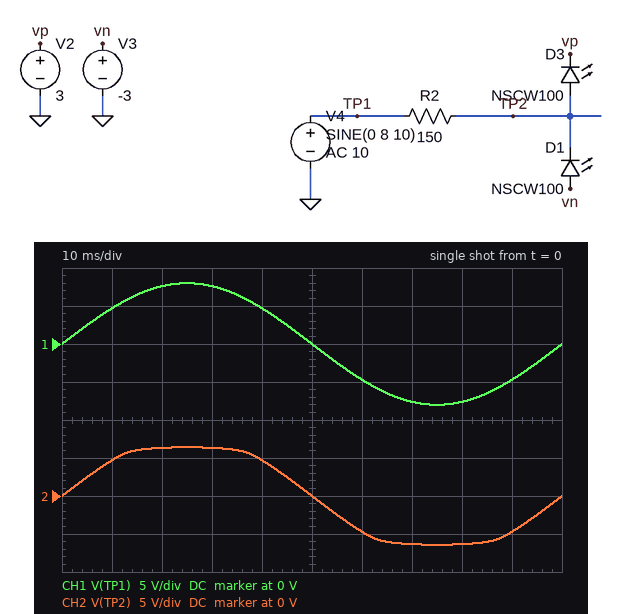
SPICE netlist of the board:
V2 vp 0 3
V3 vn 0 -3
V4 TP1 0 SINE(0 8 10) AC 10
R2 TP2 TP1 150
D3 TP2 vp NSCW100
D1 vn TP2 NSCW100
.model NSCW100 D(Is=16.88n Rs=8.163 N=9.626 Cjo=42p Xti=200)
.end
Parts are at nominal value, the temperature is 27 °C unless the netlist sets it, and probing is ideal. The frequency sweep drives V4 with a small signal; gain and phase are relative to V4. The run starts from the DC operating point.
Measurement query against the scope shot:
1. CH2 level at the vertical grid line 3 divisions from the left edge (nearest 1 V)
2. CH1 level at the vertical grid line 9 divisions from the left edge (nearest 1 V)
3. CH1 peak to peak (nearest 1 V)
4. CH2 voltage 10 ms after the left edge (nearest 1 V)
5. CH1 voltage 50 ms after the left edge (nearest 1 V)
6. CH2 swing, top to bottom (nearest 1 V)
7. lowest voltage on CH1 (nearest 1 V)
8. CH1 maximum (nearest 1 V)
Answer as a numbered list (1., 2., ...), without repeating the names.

1. 6 V
2. -5 V
3. 16 V
4. 5 V
5. 0 V
6. 13 V
7. -8 V
8. 8 V
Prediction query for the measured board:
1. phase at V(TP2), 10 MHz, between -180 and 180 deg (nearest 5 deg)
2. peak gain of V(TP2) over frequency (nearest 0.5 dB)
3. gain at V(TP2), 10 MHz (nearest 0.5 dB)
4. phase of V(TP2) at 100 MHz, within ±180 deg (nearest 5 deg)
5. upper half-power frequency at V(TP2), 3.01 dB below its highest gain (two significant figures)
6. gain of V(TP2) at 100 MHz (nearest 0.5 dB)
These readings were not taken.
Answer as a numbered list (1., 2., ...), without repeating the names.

1. -20 deg
2. 0 dB
3. -0.5 dB
4. -70 deg
5. 25 MHz
6. -12.5 dB
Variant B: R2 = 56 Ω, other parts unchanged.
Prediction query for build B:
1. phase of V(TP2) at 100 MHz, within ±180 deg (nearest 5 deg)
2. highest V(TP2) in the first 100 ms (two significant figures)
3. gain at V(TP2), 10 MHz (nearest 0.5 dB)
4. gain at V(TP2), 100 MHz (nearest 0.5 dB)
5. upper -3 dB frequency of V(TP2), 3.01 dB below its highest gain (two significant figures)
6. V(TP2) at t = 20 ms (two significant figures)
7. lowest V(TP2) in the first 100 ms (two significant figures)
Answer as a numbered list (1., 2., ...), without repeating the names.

1. -50 deg
2. 6.7 V
3. 0 dB
4. -5.5 dB
5. 63 MHz
6. 6.6 V
7. -6.7 V
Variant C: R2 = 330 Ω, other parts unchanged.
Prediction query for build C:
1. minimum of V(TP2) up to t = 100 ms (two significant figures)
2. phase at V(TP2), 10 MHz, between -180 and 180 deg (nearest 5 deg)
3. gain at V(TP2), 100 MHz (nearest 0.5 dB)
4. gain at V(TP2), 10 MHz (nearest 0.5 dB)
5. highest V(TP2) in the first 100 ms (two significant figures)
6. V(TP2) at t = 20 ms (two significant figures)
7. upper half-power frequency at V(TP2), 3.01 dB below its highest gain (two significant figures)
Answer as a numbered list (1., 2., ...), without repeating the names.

1. -6.2 V
2. -40 deg
3. -19.0 dB
4. -2.5 dB
5. 6.2 V
6. 6.1 V
7. 11 MHz
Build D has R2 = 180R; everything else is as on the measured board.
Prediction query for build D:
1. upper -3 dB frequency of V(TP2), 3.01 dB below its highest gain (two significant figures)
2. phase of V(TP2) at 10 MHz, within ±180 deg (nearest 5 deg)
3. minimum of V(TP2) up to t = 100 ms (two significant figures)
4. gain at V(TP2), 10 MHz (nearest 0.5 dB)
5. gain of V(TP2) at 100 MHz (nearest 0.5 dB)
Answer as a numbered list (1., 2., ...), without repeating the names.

1. 21 MHz
2. -25 deg
3. -6.4 V
4. -1.0 dB
5. -14.0 dB
